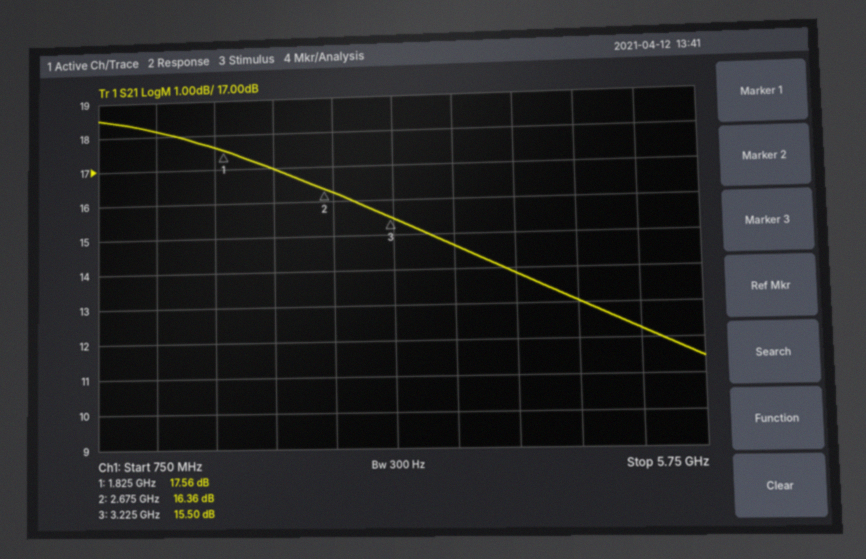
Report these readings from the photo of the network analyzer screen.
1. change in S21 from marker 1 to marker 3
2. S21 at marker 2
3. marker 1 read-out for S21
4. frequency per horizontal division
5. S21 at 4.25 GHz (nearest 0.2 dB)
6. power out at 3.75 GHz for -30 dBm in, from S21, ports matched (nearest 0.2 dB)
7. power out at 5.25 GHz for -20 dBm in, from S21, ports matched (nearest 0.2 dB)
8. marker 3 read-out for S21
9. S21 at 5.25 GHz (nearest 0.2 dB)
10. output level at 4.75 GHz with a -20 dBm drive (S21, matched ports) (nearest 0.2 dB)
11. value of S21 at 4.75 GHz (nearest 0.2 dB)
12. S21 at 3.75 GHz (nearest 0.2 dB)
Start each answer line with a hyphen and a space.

- -2.06 dB
- 16.36 dB
- 17.56 dB
- 500 MHz
- 13.8 dB
- -15.4 dBm
- -7.8 dBm
- 15.50 dB
- 12.2 dB
- -7.0 dBm
- 13.0 dB
- 14.6 dB
